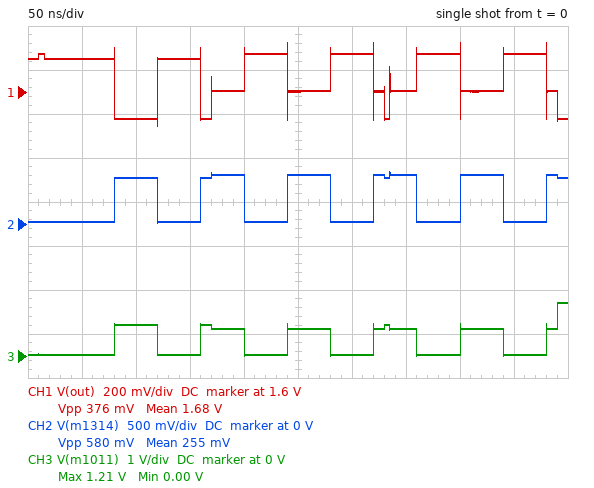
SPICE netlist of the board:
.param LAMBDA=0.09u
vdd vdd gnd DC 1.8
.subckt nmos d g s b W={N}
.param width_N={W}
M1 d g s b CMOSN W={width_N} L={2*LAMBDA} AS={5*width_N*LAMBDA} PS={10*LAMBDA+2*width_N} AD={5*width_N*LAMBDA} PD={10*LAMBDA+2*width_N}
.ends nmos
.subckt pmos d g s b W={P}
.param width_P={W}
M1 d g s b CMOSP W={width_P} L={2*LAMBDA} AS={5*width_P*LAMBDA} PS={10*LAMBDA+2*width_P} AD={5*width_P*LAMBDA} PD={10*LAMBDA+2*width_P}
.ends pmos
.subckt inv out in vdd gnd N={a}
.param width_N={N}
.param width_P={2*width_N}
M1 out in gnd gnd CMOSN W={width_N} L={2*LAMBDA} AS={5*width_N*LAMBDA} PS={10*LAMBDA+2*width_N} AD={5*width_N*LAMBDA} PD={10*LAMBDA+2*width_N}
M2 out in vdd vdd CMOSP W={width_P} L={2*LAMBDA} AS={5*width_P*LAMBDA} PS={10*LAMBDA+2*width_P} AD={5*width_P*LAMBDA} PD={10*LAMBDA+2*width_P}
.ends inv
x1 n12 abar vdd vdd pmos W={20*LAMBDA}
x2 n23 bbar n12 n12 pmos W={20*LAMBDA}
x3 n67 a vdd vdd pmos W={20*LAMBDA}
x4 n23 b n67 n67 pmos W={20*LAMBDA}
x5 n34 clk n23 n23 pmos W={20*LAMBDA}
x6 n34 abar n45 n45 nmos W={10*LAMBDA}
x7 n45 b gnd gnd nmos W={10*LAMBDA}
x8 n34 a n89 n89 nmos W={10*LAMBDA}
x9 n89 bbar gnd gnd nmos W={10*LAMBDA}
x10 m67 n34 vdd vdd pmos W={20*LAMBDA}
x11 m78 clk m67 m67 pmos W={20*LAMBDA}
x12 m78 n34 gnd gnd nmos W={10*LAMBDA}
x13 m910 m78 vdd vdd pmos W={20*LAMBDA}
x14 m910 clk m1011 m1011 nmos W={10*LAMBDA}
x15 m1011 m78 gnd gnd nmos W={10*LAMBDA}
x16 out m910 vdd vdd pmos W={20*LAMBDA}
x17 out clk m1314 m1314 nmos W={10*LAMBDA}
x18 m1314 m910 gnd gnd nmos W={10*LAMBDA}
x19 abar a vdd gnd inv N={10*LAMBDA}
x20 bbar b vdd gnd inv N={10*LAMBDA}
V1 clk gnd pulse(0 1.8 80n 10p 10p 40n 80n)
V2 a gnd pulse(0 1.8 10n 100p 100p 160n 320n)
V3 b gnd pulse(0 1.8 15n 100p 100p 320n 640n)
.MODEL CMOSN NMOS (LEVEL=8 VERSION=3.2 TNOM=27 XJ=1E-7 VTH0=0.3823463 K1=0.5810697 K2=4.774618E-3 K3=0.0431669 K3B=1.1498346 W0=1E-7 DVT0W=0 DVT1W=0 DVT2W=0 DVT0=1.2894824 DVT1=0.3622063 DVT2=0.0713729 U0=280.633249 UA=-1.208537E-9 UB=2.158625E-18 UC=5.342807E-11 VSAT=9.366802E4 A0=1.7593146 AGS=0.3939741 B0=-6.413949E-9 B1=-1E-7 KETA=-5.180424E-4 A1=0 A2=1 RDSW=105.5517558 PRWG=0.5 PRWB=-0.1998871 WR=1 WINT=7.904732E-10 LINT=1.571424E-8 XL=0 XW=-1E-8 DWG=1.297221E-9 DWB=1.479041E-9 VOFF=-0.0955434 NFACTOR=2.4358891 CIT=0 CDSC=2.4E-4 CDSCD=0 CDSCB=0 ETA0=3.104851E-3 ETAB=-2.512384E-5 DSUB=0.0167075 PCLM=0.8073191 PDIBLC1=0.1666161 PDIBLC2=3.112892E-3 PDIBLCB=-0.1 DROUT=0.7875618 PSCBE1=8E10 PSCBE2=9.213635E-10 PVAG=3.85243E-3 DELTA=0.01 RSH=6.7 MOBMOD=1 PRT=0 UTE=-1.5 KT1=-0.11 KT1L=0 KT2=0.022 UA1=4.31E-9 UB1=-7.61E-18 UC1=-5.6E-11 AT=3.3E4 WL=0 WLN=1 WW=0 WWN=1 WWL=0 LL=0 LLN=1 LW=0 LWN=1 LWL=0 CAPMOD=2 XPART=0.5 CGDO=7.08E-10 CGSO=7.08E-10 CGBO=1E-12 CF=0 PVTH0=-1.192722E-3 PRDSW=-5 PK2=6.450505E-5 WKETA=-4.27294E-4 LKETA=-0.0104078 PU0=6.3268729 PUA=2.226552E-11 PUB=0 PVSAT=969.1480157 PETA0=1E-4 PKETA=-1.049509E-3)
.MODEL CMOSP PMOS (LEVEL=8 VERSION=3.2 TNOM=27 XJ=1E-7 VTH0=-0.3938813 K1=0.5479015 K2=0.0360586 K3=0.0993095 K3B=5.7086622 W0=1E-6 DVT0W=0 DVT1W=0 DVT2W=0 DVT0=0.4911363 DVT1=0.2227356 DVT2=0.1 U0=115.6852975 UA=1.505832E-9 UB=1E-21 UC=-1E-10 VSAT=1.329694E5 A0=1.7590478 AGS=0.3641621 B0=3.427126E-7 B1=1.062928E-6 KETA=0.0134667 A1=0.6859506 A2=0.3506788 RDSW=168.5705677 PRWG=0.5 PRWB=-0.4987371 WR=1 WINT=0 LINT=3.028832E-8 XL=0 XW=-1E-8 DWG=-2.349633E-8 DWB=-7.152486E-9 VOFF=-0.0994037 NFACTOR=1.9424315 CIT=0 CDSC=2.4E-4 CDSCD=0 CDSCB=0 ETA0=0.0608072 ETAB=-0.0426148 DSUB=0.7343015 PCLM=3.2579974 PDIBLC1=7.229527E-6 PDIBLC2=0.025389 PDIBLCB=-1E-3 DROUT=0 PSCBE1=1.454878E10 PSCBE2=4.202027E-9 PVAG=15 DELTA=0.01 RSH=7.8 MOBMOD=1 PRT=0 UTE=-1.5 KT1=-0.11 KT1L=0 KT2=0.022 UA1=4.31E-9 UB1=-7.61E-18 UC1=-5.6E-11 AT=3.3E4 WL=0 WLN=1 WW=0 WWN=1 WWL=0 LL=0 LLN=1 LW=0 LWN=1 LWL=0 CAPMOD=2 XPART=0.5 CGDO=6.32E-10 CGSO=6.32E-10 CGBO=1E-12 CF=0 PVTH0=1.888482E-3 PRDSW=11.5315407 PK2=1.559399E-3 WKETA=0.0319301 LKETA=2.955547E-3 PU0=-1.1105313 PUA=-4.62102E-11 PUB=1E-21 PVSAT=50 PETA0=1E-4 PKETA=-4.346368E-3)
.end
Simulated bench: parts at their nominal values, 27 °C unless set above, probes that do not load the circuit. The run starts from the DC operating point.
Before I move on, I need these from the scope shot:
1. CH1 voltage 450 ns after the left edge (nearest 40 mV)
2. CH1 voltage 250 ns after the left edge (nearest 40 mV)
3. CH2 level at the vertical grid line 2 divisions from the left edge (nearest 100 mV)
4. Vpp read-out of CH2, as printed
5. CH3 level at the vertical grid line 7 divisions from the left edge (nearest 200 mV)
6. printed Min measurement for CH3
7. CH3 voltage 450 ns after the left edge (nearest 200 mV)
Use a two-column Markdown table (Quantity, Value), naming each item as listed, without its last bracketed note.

| Quantity | Value |
|---|---|
| CH1 voltage 450 ns after the left edge | 1.76 V |
| CH1 voltage 250 ns after the left edge | 1.60 V |
| CH2 level at the vertical grid line 2 divisions from the left edge | 500 mV |
| Vpp read-out of CH2, as printed | 580 mV |
| CH3 level at the vertical grid line 7 divisions from the left edge | 600 mV |
| printed Min measurement for CH3 | 0.00 V |
| CH3 voltage 450 ns after the left edge | 0 V |
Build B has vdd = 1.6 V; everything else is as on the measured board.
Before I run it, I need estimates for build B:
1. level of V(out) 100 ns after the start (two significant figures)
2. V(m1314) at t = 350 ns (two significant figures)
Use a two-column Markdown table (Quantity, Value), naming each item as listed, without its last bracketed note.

| Quantity | Value |
|---|---|
| level of V(out) 100 ns after the start | 1.3 V |
| V(m1314) at t = 350 ns | 520 mV |
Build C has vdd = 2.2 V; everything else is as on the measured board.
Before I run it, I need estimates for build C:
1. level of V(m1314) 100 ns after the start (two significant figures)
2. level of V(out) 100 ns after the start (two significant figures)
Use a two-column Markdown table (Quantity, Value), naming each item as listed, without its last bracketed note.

| Quantity | Value |
|---|---|
| level of V(m1314) 100 ns after the start | 550 mV |
| level of V(out) 100 ns after the start | 1.8 V |
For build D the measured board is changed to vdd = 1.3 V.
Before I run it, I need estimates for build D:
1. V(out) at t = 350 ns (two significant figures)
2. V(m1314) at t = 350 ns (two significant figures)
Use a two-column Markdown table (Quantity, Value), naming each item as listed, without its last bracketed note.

| Quantity | Value |
|---|---|
| V(out) at t = 350 ns | 1.1 V |
| V(m1314) at t = 350 ns | 520 mV |
